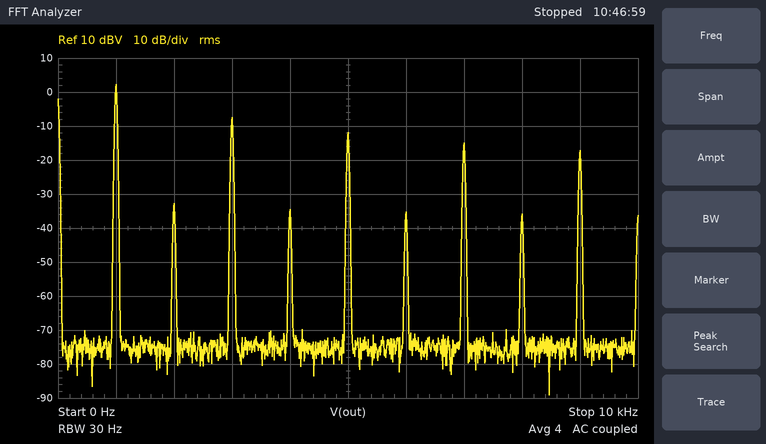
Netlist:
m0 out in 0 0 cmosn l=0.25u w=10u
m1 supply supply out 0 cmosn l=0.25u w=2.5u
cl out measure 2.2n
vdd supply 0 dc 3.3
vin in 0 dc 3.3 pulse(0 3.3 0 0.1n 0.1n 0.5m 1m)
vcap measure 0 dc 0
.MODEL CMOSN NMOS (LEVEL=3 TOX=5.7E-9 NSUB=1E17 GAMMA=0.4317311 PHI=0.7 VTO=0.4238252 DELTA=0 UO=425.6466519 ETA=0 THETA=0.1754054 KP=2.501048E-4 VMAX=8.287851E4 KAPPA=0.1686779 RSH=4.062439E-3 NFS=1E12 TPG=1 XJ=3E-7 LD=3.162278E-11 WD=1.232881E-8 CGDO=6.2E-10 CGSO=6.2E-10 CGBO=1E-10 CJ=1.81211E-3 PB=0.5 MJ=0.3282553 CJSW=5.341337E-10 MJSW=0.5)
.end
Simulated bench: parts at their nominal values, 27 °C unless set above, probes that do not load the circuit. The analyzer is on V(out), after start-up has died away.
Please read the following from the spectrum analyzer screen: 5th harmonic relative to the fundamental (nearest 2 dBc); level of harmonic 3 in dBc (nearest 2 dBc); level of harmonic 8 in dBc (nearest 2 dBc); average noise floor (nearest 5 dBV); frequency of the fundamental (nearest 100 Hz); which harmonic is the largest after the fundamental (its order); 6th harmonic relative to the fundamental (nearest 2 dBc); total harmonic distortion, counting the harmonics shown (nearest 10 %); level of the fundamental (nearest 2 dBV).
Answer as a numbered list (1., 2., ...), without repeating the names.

1. -14 dBc
2. -10 dBc
3. -38 dBc
4. -75 dBV
5. 1.0 kHz
6. 3
7. -38 dBc
8. 40 %
9. 2 dBV
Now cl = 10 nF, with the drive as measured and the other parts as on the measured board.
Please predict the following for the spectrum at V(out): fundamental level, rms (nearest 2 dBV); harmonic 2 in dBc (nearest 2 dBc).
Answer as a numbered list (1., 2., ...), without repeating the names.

1. 2 dBV
2. -26 dBc
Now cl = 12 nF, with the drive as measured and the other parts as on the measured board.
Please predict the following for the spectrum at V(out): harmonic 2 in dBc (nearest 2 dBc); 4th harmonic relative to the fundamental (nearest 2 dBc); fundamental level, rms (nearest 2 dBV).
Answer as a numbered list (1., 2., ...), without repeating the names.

1. -24 dBc
2. -26 dBc
3. 2 dBV
